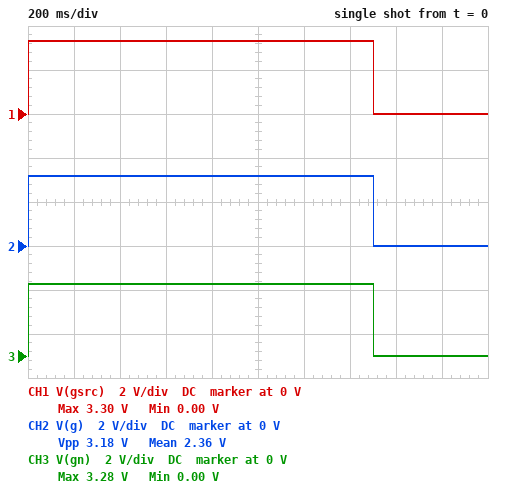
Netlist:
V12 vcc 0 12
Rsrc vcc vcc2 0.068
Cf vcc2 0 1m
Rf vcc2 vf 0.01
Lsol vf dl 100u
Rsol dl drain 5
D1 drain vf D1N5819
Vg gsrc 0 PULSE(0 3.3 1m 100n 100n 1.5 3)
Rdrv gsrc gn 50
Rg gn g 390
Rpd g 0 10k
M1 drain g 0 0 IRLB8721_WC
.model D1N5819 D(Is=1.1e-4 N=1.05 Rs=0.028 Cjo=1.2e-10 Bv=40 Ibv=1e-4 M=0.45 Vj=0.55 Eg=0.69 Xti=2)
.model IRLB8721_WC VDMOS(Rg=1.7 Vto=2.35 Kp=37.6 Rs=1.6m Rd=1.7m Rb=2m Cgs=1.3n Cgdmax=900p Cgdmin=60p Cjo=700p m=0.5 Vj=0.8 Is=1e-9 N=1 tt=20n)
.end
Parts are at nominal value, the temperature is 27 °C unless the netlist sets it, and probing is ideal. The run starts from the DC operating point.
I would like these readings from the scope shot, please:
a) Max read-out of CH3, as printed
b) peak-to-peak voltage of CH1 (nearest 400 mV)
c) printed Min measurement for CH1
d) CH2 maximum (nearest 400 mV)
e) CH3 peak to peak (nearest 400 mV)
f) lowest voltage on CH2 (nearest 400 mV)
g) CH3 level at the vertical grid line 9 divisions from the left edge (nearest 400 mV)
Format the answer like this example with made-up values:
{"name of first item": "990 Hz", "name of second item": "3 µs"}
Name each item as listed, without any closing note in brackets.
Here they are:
{"Max read-out of CH3, as printed": "3.28 V", "peak-to-peak voltage of CH1": "3.2 V", "printed Min measurement for CH1": "0.00 V", "CH2 maximum": "3.2 V", "CH3 peak to peak": "3.2 V", "lowest voltage on CH2": "0 V", "CH3 level at the vertical grid line 9 divisions from the left edge": "0 V"}
